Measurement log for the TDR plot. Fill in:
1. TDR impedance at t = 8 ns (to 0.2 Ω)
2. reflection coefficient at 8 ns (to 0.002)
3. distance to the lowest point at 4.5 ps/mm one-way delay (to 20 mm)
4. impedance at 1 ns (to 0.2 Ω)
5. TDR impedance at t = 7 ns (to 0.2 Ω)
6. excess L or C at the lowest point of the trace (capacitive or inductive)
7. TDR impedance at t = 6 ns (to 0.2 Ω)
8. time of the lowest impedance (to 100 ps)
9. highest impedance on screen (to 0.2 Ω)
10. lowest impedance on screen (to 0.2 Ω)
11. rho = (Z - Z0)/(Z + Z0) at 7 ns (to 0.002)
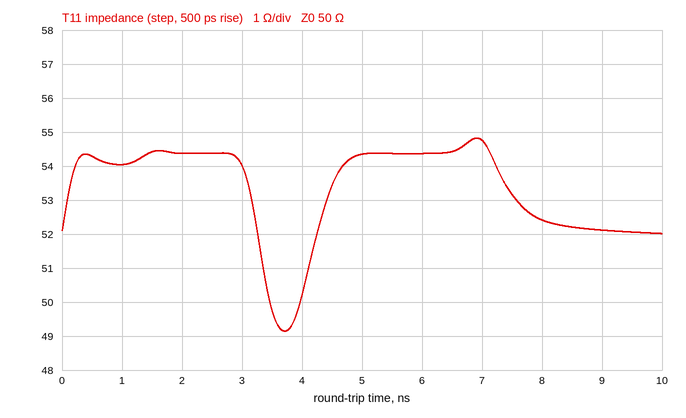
52.4 Ω
+0.024
420 mm
54.0 Ω
54.8 Ω
capacitive
54.4 Ω
3.7 ns
54.8 Ω
49.2 Ω
+0.046
